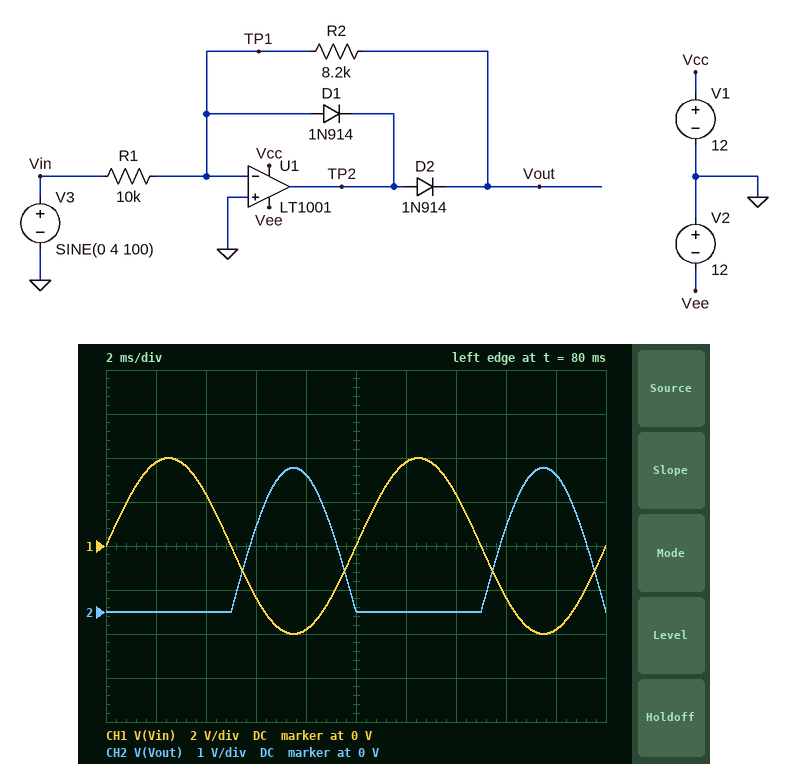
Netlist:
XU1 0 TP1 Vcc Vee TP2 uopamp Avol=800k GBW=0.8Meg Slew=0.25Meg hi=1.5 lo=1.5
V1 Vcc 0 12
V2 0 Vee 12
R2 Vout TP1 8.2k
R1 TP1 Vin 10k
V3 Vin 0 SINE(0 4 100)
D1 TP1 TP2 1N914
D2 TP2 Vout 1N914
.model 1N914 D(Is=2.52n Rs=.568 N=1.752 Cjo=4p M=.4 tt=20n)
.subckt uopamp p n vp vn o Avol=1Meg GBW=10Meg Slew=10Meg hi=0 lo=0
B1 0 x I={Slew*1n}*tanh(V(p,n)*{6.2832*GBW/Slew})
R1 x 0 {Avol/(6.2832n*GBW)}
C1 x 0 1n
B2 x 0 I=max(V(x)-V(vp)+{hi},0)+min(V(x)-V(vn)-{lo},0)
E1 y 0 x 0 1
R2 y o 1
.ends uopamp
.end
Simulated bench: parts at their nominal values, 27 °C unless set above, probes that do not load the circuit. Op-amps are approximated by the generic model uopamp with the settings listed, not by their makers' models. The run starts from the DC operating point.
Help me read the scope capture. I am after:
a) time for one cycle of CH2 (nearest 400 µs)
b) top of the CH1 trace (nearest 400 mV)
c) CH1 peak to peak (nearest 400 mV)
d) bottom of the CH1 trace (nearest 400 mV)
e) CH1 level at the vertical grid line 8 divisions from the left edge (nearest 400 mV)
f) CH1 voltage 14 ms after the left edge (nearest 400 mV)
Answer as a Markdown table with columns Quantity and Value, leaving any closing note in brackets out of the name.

| Quantity | Value |
|---|---|
| time for one cycle of CH2 | 10.0 ms |
| top of the CH1 trace | 4.0 V |
| CH1 peak to peak | 8.0 V |
| bottom of the CH1 trace | -4.0 V |
| CH1 level at the vertical grid line 8 divisions from the left edge | -2.4 V |
| CH1 voltage 14 ms after the left edge | 2.4 V |
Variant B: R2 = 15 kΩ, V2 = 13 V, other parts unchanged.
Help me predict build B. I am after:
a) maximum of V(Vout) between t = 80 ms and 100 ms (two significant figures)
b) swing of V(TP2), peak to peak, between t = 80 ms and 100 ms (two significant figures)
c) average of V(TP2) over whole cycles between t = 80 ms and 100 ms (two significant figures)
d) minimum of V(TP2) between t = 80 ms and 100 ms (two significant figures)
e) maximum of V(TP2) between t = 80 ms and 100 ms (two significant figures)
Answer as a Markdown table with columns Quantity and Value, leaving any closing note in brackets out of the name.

| Quantity | Value |
|---|---|
| maximum of V(Vout) between t = 80 ms and 100 ms | 6.0 V |
| swing of V(TP2), peak to peak, between t = 80 ms and 100 ms | 7.1 V |
| average of V(TP2) over whole cycles between t = 80 ms and 100 ms | 1.9 V |
| minimum of V(TP2) between t = 80 ms and 100 ms | -540 mV |
| maximum of V(TP2) between t = 80 ms and 100 ms | 6.5 V |
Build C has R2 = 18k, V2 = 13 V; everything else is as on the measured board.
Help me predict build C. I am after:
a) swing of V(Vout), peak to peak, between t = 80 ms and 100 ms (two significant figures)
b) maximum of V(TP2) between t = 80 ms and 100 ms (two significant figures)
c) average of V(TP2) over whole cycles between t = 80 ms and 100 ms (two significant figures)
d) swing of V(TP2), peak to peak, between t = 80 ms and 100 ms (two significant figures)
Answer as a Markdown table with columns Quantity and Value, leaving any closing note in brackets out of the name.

| Quantity | Value |
|---|---|
| swing of V(Vout), peak to peak, between t = 80 ms and 100 ms | 7.2 V |
| maximum of V(TP2) between t = 80 ms and 100 ms | 7.7 V |
| average of V(TP2) over whole cycles between t = 80 ms and 100 ms | 2.3 V |
| swing of V(TP2), peak to peak, between t = 80 ms and 100 ms | 8.3 V |
